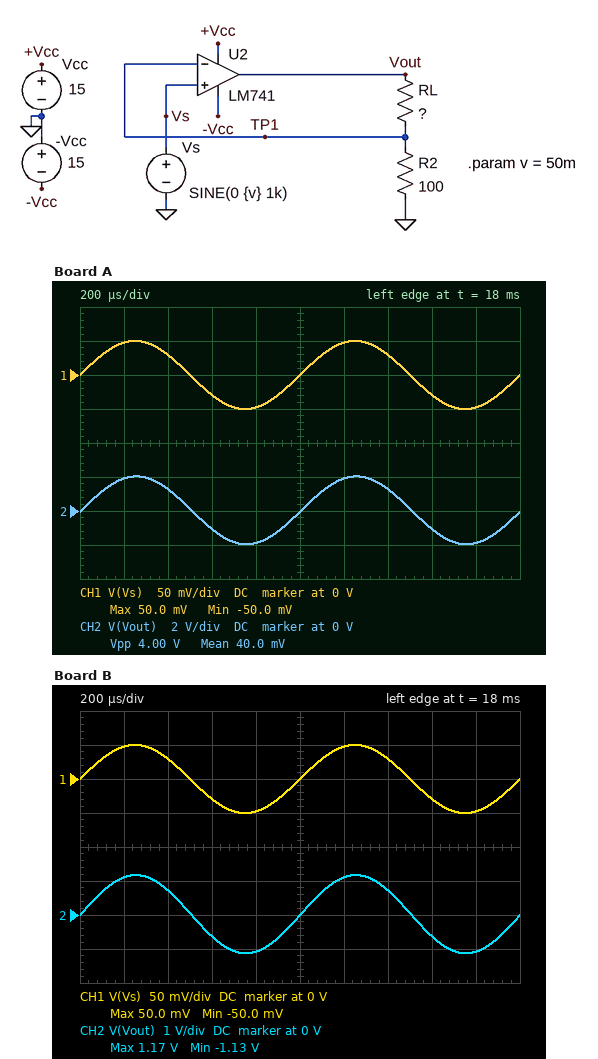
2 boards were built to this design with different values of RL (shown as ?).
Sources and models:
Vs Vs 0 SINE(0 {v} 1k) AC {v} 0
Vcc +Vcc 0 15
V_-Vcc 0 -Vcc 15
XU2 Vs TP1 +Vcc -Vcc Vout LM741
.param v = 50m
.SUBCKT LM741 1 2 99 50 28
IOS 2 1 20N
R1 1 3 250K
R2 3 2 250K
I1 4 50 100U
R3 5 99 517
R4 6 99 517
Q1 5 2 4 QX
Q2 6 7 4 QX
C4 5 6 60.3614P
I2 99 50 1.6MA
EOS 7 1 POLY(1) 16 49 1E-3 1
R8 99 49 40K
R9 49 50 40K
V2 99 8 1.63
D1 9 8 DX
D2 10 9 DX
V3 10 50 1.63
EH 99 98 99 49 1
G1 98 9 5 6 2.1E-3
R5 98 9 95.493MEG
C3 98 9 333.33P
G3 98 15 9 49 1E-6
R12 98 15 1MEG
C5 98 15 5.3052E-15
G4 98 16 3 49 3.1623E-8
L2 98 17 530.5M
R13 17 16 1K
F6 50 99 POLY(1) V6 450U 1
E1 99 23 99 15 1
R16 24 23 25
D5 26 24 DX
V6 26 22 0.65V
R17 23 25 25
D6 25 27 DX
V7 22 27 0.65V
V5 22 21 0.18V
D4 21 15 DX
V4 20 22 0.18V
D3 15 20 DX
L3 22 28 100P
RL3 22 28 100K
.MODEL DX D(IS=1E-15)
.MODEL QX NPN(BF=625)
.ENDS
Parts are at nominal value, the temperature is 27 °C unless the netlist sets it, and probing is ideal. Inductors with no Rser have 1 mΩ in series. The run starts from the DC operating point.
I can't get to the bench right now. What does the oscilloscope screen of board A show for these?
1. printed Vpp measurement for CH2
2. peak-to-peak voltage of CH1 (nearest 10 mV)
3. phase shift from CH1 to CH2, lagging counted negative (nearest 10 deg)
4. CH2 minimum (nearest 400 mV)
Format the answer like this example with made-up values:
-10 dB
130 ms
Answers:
4.00 V
100 mV
0 deg
-2.0 V
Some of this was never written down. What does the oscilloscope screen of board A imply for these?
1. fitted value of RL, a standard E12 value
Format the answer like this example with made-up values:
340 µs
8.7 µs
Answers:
3.9 kΩ
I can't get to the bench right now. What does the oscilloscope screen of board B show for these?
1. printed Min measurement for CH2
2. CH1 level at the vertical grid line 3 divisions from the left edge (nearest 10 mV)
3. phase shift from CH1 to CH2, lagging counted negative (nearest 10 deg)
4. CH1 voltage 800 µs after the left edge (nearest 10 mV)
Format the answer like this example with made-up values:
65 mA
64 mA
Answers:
-1.13 V
-30 mV
0 deg
-50 mV
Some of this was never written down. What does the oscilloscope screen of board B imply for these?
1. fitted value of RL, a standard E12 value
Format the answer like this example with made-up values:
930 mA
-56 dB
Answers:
2.2 kΩ
